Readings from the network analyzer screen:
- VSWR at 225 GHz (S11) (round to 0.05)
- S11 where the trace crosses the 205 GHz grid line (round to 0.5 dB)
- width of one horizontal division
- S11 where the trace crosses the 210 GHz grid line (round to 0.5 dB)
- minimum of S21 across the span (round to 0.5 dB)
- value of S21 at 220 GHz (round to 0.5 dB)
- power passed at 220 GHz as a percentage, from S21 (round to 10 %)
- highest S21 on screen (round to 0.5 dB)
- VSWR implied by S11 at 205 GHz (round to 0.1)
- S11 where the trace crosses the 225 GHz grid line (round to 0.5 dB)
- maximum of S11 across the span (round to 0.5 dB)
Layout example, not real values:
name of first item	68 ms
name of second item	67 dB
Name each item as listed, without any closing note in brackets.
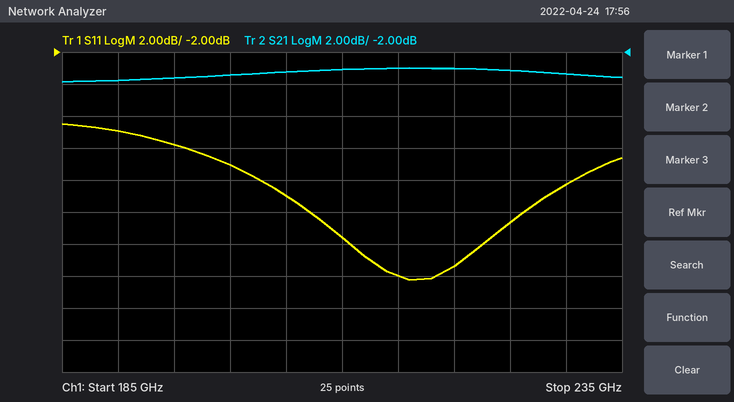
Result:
VSWR at 225 GHz (S11)	1.60
S11 where the trace crosses the 205 GHz grid line	-11.0 dB
width of one horizontal division	5 GHz
S11 where the trace crosses the 210 GHz grid line	-13.5 dB
minimum of S21 across the span	-4.0 dB
value of S21 at 220 GHz	-3.0 dB
power passed at 220 GHz as a percentage, from S21	50 %
highest S21 on screen	-3.0 dB
VSWR implied by S11 at 205 GHz	1.8
S11 where the trace crosses the 225 GHz grid line	-12.5 dB
maximum of S11 across the span	-6.5 dB
